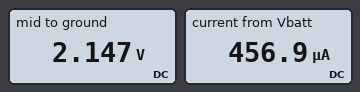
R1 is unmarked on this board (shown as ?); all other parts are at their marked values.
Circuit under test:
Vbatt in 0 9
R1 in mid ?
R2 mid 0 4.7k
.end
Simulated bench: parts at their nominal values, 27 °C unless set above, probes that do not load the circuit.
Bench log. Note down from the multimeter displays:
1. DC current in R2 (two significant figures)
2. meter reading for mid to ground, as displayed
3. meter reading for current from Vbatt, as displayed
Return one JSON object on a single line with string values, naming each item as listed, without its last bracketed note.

{"DC current in R2": "460 µA", "meter reading for mid to ground, as displayed": "2.147 V", "meter reading for current from Vbatt, as displayed": "456.9 µA"}
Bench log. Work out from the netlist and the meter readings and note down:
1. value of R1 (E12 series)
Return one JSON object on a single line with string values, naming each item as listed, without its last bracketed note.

{"value of R1": "15 kΩ"}
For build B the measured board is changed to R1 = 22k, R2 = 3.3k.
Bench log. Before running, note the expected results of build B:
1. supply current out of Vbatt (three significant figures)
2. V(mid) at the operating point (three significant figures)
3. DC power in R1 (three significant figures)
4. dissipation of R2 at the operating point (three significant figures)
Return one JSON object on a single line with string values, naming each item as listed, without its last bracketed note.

{"supply current out of Vbatt": "356 µA", "V(mid) at the operating point": "1.17 V", "DC power in R1": "2.78 mW", "dissipation of R2 at the operating point": "418 µW"}
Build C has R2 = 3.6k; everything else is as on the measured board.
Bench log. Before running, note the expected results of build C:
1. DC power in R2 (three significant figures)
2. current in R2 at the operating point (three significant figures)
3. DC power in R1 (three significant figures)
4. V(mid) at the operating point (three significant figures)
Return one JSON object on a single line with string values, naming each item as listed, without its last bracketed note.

{"DC power in R2": "843 µW", "current in R2 at the operating point": "484 µA", "DC power in R1": "3.51 mW", "V(mid) at the operating point": "1.74 V"}
